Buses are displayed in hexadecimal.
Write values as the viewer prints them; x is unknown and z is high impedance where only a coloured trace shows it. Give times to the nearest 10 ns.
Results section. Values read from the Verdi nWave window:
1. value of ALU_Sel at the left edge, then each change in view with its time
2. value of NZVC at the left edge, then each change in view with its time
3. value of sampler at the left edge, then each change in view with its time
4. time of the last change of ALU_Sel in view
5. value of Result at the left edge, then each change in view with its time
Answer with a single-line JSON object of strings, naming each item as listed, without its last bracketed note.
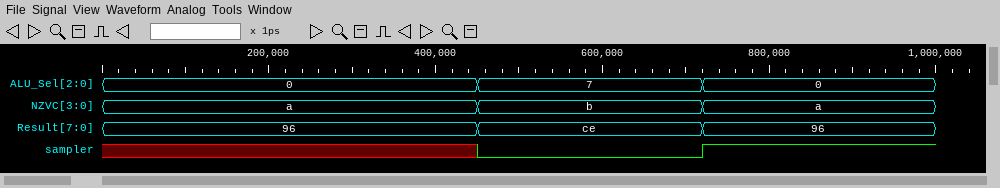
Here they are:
{"value of ALU_Sel at the left edge, then each change in view with its time": "0, 7 at 450 ns, 0 at 720 ns", "value of NZVC at the left edge, then each change in view with its time": "a, b at 450 ns, a at 720 ns", "value of sampler at the left edge, then each change in view with its time": "x, 0 at 450 ns, 1 at 720 ns", "time of the last change of ALU_Sel in view": "720 ns", "value of Result at the left edge, then each change in view with its time": "96, ce at 450 ns, 96 at 720 ns"}
